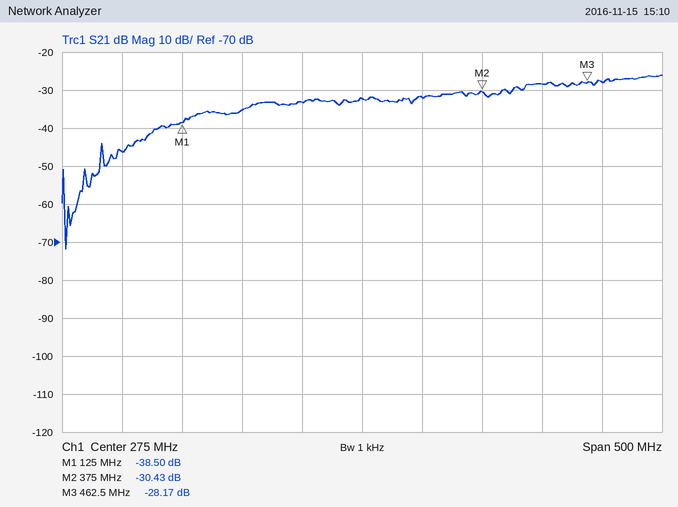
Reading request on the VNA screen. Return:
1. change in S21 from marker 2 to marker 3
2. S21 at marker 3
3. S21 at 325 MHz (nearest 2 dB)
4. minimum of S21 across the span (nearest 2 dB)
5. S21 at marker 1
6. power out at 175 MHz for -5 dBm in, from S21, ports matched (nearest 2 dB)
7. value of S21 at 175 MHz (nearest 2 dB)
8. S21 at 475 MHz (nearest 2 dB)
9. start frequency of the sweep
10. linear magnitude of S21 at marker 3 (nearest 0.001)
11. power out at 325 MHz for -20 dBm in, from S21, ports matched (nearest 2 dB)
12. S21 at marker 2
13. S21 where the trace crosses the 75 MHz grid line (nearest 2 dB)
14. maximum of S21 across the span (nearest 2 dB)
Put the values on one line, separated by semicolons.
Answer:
2.26 dB; -28.17 dB; -32 dB; -72 dB; -38.50 dB; -40 dBm; -36 dB; -28 dB; 25 MHz; 0.039; -52 dBm; -30.43 dB; -46 dB; -26 dB
